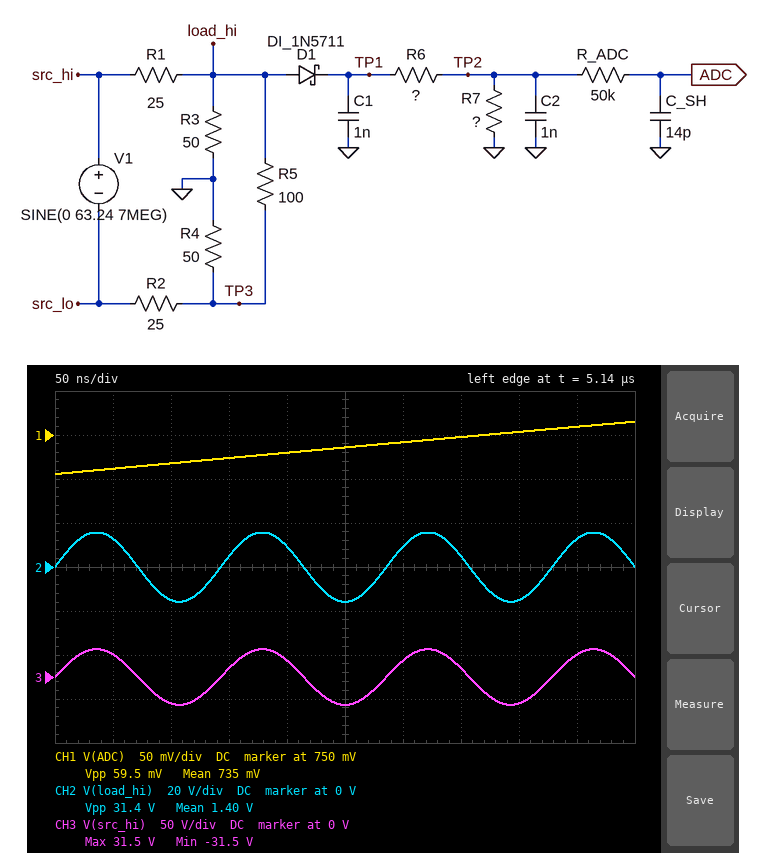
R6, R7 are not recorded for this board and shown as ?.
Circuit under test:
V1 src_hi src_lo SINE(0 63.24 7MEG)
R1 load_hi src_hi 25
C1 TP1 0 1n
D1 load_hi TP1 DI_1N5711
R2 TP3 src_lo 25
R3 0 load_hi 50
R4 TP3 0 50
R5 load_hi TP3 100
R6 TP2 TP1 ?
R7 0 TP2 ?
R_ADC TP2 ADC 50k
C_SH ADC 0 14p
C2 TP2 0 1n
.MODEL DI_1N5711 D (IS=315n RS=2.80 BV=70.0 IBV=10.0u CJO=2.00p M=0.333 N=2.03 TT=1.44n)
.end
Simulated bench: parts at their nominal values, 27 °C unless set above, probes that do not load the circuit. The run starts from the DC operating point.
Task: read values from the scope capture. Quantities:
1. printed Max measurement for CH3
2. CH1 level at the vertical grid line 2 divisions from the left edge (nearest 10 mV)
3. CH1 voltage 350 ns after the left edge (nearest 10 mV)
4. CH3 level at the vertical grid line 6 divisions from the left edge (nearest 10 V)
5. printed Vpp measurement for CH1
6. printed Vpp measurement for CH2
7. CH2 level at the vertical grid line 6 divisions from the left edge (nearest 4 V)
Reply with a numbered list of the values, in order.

1. 31.5 V
2. 720 mV
3. 750 mV
4. 20 V
5. 59.5 mV
6. 31.4 V
7. 8 V
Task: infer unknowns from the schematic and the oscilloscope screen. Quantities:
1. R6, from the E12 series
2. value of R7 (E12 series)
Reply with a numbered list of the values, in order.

1. 68 kΩ
2. 8.2 kΩ
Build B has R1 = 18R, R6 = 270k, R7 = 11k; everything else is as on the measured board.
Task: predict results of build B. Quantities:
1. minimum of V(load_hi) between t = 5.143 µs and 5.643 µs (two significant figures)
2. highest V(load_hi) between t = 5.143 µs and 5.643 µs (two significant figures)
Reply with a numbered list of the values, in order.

1. -17 V
2. 17 V
